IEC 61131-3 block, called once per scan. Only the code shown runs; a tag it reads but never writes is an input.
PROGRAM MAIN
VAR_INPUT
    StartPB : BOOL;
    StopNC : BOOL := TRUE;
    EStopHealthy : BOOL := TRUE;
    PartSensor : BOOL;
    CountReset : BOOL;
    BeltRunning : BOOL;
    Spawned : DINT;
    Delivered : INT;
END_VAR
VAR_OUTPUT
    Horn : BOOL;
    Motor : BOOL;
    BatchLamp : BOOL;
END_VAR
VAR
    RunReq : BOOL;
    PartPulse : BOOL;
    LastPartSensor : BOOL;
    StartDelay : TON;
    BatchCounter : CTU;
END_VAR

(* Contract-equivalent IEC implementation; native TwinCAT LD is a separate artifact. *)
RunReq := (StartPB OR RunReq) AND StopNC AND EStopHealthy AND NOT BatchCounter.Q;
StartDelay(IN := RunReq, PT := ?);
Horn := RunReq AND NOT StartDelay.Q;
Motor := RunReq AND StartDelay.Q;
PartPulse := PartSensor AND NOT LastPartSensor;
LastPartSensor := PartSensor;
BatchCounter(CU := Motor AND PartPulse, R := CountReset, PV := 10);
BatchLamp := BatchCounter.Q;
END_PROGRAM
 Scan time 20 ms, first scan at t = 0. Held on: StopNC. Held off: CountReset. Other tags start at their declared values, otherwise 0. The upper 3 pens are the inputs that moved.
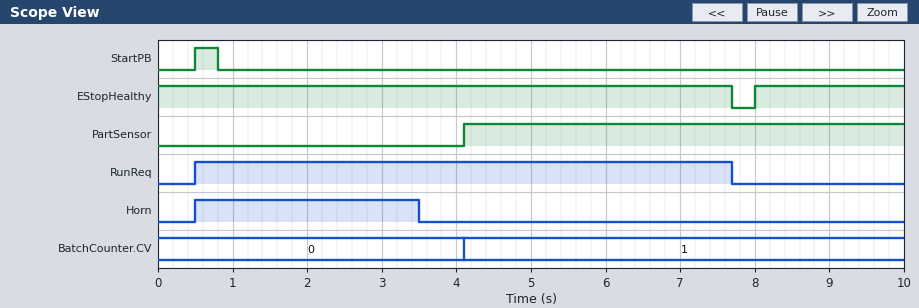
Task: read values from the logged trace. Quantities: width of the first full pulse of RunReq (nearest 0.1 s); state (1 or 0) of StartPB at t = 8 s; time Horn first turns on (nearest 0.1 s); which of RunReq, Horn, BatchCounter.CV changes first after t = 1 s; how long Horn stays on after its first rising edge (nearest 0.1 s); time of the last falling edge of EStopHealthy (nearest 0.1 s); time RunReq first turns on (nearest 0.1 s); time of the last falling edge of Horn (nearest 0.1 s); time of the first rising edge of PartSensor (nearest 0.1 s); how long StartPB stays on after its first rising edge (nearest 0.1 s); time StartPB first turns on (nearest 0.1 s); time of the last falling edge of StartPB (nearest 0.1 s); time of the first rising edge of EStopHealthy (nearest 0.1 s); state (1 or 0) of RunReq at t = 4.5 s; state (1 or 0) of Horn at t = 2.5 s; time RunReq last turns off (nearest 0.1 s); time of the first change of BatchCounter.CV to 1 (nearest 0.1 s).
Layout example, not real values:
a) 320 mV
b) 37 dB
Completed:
a) 7.2 s
b) 0
c) 0.5 s
d) Horn
e) 3.0 s
f) 7.7 s
g) 0.5 s
h) 3.5 s
i) 4.1 s
j) 0.3 s
k) 0.5 s
l) 0.8 s
m) 8.0 s
n) 1
o) 1
p) 7.7 s
q) 4.1 s
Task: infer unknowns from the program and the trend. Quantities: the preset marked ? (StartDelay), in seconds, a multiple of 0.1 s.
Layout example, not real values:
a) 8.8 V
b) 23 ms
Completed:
a) 3.0 s
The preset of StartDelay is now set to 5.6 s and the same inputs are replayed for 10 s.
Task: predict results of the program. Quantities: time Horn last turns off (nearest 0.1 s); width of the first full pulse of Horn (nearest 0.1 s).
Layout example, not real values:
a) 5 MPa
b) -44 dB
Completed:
a) 6.1 s
b) 5.6 s
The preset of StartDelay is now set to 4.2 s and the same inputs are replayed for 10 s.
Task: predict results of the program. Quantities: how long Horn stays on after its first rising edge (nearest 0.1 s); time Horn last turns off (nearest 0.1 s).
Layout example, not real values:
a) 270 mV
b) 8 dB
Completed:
a) 4.2 s
b) 4.7 s
